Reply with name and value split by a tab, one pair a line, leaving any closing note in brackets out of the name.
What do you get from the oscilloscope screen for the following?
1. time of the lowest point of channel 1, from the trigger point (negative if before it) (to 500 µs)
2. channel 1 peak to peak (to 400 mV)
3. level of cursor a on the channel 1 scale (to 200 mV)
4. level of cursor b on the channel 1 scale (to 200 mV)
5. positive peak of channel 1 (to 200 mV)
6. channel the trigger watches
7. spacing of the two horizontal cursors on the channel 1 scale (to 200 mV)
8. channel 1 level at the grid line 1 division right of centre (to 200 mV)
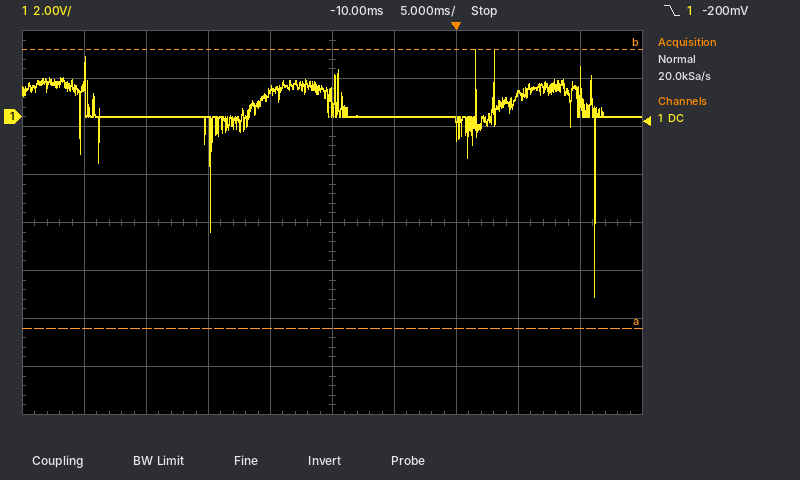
time of the lowest point of channel 1, from the trigger point (negative if before it)	+11.0 ms
channel 1 peak to peak	10.4 V
level of cursor a on the channel 1 scale	-8.8 V
level of cursor b on the channel 1 scale	2.8 V
positive peak of channel 1	2.8 V
channel the trigger watches	channel 1
spacing of the two horizontal cursors on the channel 1 scale	11.6 V
channel 1 level at the grid line 1 division right of centre	0.0 V
